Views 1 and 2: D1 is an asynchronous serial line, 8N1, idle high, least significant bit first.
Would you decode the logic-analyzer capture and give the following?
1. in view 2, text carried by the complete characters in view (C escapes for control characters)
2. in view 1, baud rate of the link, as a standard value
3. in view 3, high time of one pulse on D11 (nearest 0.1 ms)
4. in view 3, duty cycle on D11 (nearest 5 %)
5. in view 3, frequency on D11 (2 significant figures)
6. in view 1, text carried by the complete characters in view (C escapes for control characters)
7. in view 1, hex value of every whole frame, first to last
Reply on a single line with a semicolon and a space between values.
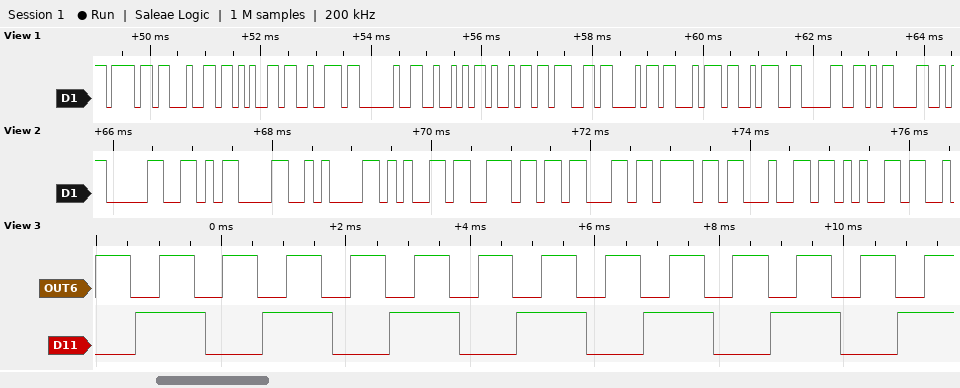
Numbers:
"0\r\nencode"; 9600 baud; 1.1 ms; 55 %; 490 Hz; "oder Right:0\r"; 6F 64 65 72 20 52 69 67 68 74 3A 30 0D
